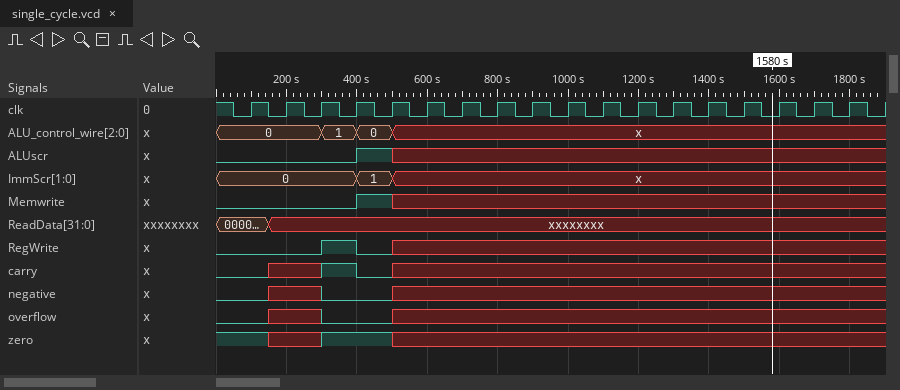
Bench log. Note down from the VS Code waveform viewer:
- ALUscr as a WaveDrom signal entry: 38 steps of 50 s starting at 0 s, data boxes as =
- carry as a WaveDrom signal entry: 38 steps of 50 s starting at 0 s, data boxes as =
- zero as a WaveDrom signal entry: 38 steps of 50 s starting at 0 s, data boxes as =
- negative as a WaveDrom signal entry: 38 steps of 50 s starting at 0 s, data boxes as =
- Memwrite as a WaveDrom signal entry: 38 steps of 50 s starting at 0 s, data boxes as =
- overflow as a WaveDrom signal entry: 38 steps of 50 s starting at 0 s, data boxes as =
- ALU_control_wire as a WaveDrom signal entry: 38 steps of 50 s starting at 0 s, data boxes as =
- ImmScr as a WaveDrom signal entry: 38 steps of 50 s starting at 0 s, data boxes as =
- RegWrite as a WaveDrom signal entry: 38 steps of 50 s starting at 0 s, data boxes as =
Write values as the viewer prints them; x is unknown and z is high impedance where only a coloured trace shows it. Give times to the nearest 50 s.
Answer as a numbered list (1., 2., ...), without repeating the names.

1. {name: 'ALUscr', wave: '0.......1.x...........................'}
2. {name: 'carry', wave: '0..x..1.0.x...........................'}
3. {name: 'zero', wave: '1..x..1...x...........................'}
4. {name: 'negative', wave: '0..x..0...x...........................'}
5. {name: 'Memwrite', wave: '0.......1.x...........................'}
6. {name: 'overflow', wave: '0..x..0...x...........................'}
7. {name: 'ALU_control_wire', wave: '=.....=.=.x...........................', data: '0 1 0'}
8. {name: 'ImmScr', wave: '=.......=.x...........................', data: '0 1'}
9. {name: 'RegWrite', wave: '0.....1.0.x...........................'}
